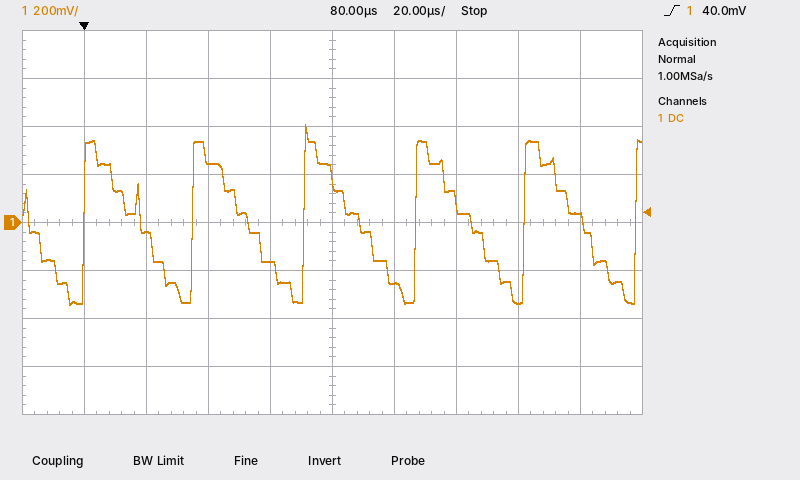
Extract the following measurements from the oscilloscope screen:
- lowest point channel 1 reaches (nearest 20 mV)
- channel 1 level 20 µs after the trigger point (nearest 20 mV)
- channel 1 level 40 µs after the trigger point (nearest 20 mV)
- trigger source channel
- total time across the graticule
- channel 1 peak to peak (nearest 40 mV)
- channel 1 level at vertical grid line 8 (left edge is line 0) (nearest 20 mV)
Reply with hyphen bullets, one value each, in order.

- -340 mV
- -40 mV
- 260 mV
- channel 1
- 200 µs
- 760 mV
- -340 mV
